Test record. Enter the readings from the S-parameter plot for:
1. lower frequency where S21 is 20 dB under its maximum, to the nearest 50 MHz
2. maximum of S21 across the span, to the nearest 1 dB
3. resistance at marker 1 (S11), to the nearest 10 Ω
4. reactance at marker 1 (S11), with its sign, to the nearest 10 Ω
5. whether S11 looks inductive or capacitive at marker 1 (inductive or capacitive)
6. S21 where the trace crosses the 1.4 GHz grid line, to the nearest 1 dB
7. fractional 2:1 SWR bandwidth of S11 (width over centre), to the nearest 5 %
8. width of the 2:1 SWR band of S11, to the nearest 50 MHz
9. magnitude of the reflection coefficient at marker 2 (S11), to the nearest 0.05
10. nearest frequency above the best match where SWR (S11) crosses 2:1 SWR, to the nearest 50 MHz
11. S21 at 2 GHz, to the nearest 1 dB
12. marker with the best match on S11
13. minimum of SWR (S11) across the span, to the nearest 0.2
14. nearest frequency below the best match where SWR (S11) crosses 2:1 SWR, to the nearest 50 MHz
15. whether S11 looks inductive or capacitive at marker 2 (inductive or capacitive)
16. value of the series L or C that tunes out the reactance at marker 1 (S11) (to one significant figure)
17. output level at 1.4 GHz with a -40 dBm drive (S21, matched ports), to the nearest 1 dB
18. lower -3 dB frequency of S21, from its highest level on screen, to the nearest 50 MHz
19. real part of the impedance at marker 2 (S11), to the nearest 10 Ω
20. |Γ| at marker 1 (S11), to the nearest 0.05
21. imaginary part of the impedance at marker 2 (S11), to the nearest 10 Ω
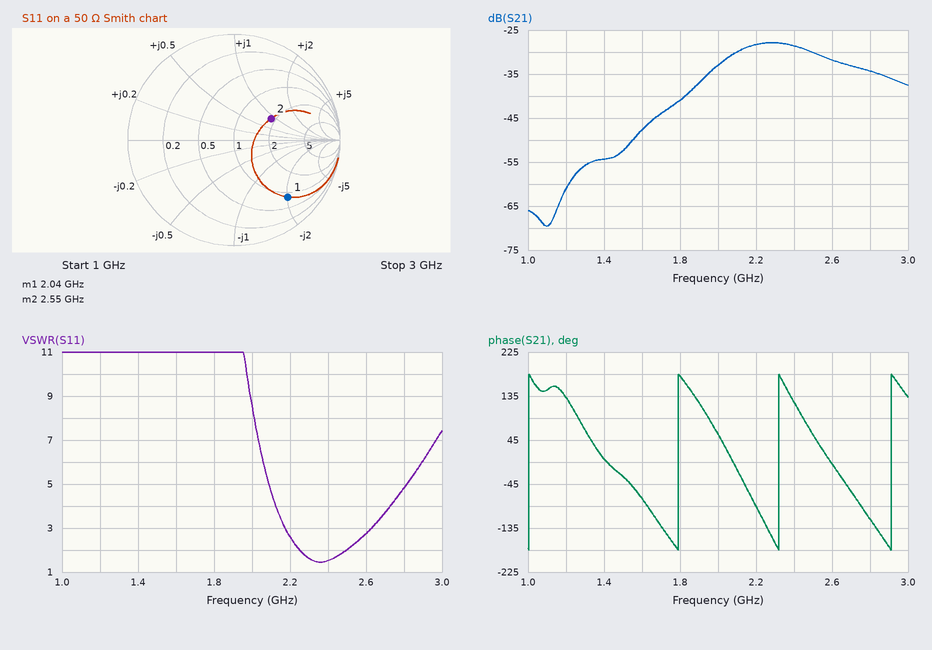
1.60 GHz
-28 dB
40 Ω
-100 Ω
capacitive
-54 dB
10 %
250 MHz
0.40
2.50 GHz
-33 dB
marker 2
1.4
2.25 GHz
inductive
8 nH
-94 dBm
2.05 GHz
90 Ω
0.75
+40 Ω
